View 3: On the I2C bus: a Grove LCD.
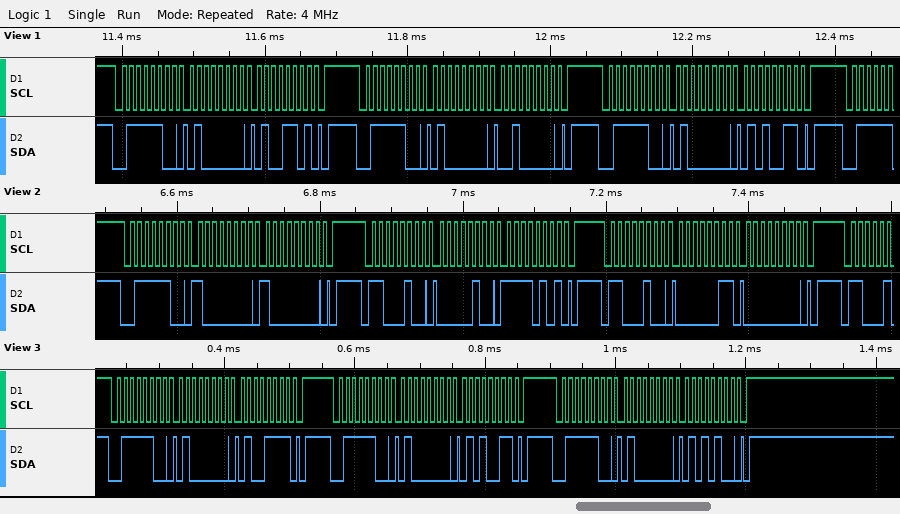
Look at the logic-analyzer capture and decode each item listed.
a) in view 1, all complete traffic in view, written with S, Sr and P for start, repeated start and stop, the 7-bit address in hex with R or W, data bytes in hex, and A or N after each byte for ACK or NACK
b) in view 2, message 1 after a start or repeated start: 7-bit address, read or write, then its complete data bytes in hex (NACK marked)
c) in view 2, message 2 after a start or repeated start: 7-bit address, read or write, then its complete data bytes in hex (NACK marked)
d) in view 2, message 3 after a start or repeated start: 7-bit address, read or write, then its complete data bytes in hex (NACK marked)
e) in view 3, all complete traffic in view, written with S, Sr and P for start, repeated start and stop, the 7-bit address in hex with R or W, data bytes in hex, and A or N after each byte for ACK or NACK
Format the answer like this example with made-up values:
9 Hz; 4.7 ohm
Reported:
S 3EW A 40 A 4D A P S 3EW A 40 A 20 A P S 3EW A 40 A 53 A P; 0x3E write: 80 80; 0x62 write: 04 F5; 0x62 write: 03 00; S 3EW A 40 A 4F A P S 3EW A 40 A 53 A P S 3EW A 40 A 54 A P
